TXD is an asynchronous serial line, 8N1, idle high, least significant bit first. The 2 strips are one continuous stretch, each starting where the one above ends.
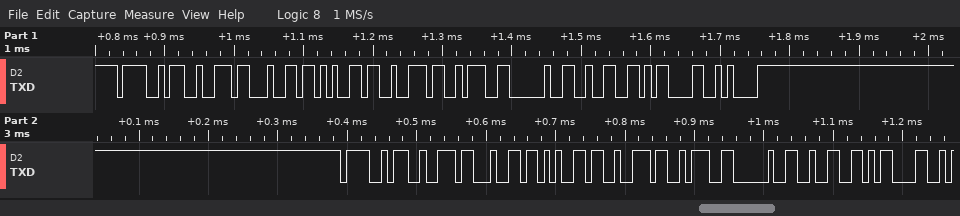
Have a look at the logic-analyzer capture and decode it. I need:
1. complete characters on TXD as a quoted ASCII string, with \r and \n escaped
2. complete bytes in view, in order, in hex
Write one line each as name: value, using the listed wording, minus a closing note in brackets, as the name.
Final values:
complete characters on TXD as a quoted ASCII string, with \r and \n escaped: "Order: 2\r\nOrder: 2\r"
complete bytes in view, in order, in hex: 4F 72 64 65 72 3A 20 32 0D 0A 4F 72 64 65 72 3A 20 32 0D
